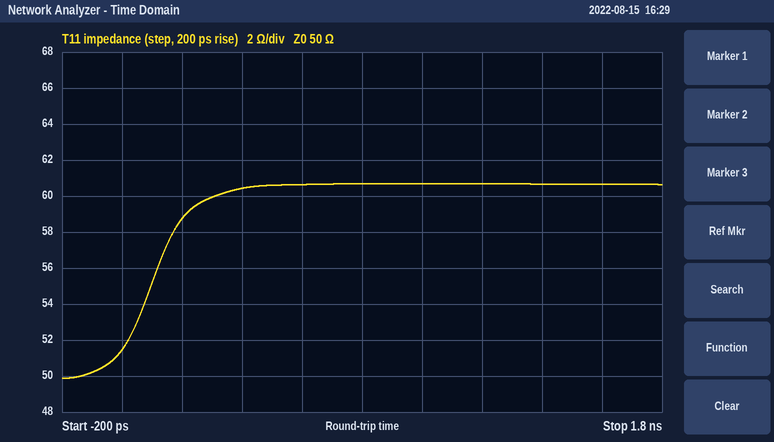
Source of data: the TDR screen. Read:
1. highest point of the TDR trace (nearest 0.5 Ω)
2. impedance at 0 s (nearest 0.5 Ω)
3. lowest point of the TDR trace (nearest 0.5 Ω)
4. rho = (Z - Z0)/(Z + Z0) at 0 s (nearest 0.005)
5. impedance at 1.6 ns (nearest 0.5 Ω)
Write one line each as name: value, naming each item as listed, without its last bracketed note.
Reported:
highest point of the TDR trace: 60.5 Ω
impedance at 0 s: 51.5 Ω
lowest point of the TDR trace: 50.0 Ω
rho = (Z - Z0)/(Z + Z0) at 0 s: +0.015
impedance at 1.6 ns: 60.5 Ω
